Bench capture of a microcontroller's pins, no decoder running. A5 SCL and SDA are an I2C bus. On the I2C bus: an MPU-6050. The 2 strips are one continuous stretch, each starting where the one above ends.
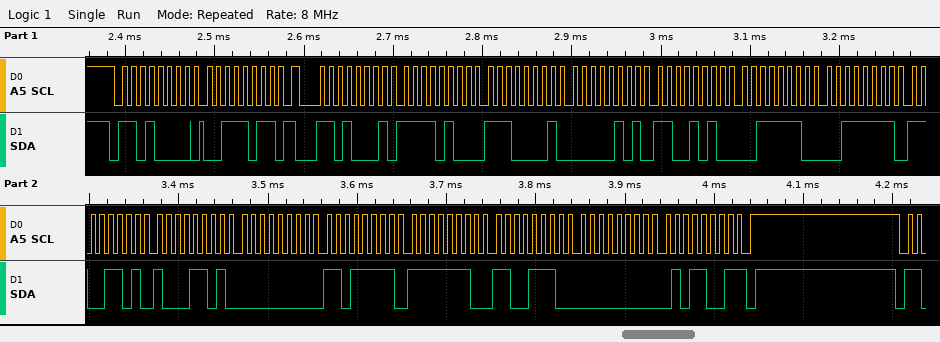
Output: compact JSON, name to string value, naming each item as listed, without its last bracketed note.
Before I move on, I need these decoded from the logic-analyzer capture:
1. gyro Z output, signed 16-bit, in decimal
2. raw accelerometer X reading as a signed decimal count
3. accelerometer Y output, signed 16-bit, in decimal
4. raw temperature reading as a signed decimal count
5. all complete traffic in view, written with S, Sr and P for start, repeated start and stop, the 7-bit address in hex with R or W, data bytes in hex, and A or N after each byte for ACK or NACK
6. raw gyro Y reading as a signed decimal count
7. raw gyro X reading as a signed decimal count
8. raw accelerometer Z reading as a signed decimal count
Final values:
{"gyro Z output, signed 16-bit, in decimal": "89", "raw accelerometer X reading as a signed decimal count": "-2847", "accelerometer Y output, signed 16-bit, in decimal": "1482", "raw temperature reading as a signed decimal count": "-12915", "all complete traffic in view, written with S, Sr and P for start, repeated start and stop, the 7-bit address in hex with R or W, data bytes in hex, and A or N after each byte for ACK or NACK": "S 68W A 3B A Sr 68R A F4 A E1 A 05 A CA A 3E A 3F A CD A 8D A 00 A DF A FE A CE A 00 A 59 N P", "raw gyro Y reading as a signed decimal count": "-306", "raw gyro X reading as a signed decimal count": "223", "raw accelerometer Z reading as a signed decimal count": "15935"}
